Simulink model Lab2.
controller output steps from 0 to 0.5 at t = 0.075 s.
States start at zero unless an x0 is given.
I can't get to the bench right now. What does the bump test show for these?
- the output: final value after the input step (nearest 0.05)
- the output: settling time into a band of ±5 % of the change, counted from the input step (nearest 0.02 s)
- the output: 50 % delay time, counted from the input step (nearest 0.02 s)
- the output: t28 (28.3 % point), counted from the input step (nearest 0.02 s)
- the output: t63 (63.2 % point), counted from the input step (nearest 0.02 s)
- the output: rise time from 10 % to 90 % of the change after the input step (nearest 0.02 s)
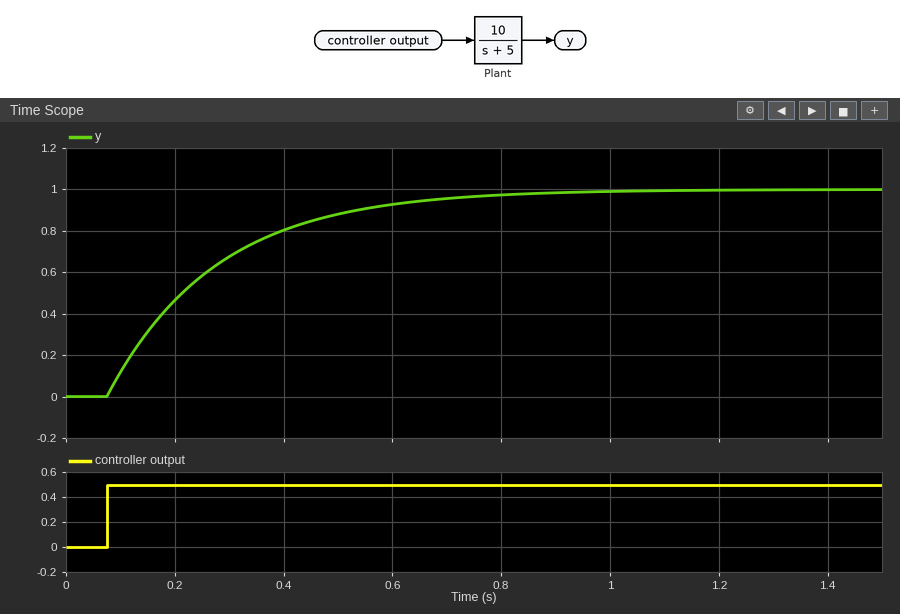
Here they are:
1.00
0.60 s
0.14 s
0.06 s
0.20 s
0.44 s
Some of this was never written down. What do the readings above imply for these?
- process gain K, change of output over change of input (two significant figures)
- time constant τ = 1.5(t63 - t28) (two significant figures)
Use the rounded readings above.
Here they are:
2.0
0.21 s
